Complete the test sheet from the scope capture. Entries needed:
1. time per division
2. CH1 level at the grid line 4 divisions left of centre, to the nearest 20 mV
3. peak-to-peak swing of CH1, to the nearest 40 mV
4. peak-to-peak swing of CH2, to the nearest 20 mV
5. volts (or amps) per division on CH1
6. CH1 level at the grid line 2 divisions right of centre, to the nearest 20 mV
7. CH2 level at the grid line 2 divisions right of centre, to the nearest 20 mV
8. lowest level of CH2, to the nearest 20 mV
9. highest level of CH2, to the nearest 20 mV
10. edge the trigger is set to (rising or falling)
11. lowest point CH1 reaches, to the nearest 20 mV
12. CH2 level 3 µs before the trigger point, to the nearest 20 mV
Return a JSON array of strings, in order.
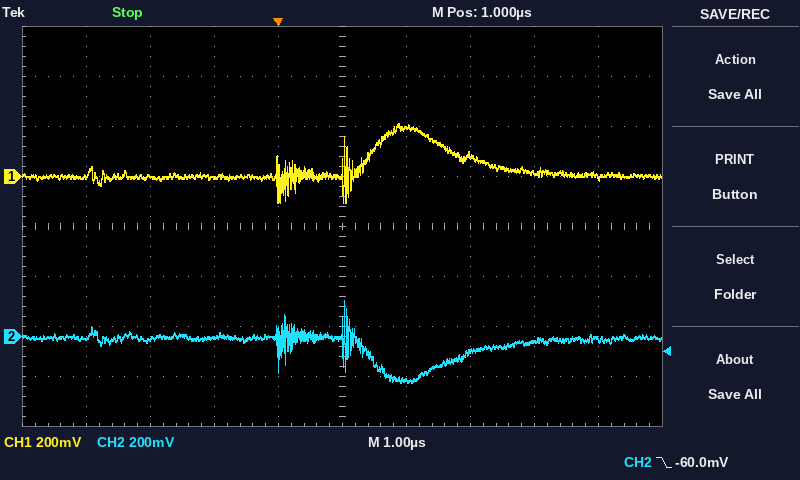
["1 µs", "0 mV", "320 mV", "320 mV", "200 mV", "80 mV", "-60 mV", "-180 mV", "140 mV", "falling", "-100 mV", "0 mV"]
